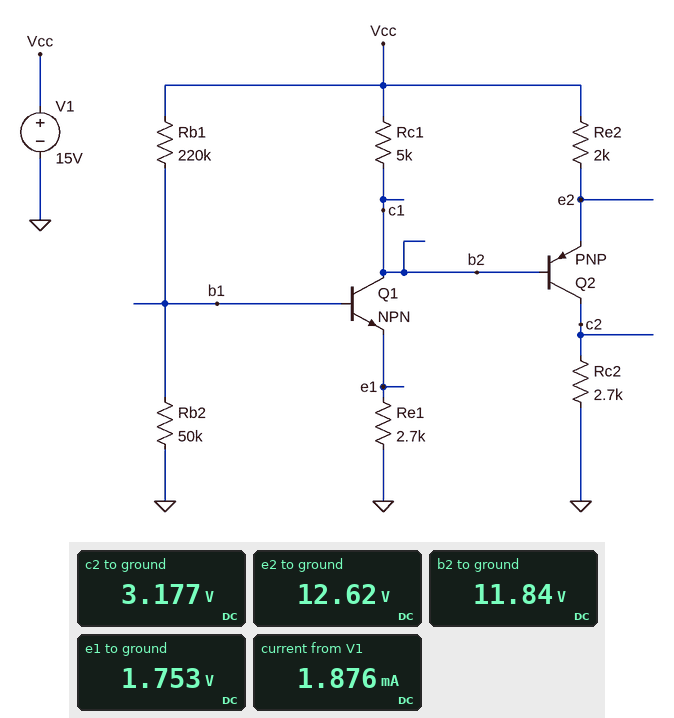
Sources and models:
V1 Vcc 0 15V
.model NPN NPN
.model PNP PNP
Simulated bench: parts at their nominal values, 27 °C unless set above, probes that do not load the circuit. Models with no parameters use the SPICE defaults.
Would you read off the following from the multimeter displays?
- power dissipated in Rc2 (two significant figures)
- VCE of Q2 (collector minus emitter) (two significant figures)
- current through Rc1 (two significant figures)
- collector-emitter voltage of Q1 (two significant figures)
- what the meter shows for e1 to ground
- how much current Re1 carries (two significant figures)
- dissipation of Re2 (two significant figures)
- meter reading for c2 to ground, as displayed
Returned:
3.7 mW
-9.4 V
630 µA
10 V
1.753 V
650 µA
2.8 mW
3.177 V
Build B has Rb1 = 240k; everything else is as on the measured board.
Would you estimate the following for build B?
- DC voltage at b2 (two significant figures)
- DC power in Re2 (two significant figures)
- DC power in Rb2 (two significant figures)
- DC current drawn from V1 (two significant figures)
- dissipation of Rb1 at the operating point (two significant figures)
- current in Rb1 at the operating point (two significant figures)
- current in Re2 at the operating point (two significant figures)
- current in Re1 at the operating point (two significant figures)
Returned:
12 V
2.2 mW
110 µW
1.7 mA
670 µW
53 µA
1.0 mA
590 µA
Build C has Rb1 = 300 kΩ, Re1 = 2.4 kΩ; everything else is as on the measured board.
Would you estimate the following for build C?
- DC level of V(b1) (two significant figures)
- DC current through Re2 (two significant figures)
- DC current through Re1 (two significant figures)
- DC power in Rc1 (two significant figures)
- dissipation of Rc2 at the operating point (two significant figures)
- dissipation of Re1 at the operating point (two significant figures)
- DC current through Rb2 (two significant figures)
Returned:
1.9 V
810 µA
490 µA
1.1 mW
1.7 mW
580 µW
39 µA
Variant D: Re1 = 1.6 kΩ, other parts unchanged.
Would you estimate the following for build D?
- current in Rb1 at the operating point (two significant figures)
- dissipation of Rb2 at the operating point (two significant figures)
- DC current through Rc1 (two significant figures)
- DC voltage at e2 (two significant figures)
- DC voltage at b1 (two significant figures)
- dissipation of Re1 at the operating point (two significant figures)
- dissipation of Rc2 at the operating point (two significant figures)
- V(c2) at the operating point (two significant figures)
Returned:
57 µA
110 µW
970 µA
11 V
2.4 V
1.6 mW
11 mW
5.4 V
